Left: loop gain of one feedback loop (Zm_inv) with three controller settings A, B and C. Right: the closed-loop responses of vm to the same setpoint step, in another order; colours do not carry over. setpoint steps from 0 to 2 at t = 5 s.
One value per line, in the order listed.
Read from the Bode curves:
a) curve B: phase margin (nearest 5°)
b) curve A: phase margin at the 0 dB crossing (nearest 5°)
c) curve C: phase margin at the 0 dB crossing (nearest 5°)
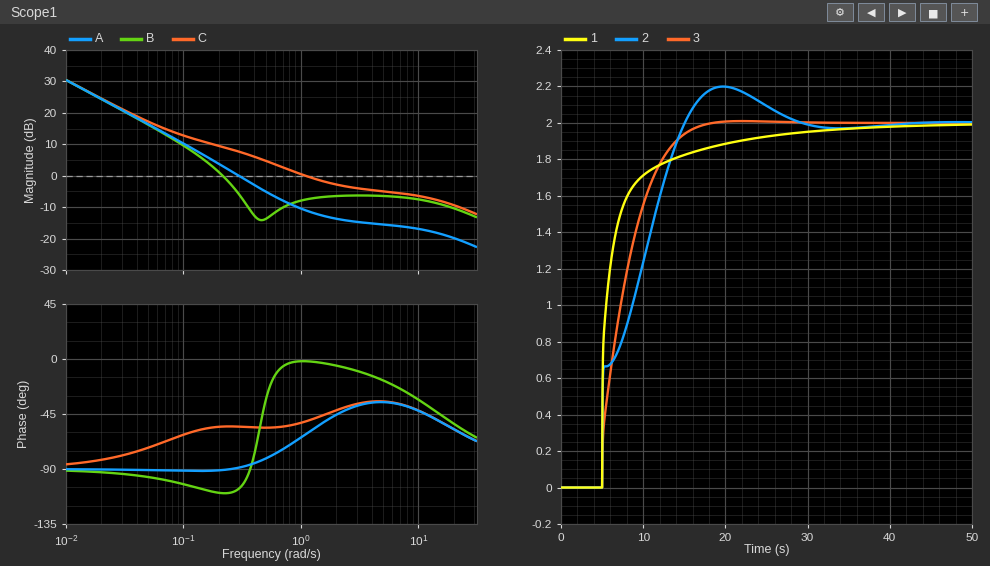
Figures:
70°
90°
130°
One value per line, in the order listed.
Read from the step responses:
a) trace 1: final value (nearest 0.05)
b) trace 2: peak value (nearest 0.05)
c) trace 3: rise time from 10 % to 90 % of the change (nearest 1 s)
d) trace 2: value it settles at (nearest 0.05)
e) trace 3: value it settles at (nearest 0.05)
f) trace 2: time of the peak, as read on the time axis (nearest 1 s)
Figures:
2.00
2.20
7 s
2.00
2.00
20 s
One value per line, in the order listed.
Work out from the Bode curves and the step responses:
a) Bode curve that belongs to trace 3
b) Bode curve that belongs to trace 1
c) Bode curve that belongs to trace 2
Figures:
A
C
B
